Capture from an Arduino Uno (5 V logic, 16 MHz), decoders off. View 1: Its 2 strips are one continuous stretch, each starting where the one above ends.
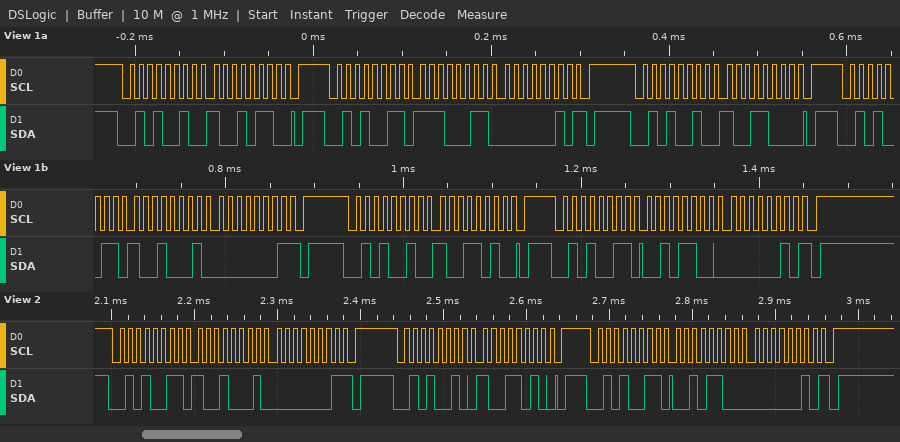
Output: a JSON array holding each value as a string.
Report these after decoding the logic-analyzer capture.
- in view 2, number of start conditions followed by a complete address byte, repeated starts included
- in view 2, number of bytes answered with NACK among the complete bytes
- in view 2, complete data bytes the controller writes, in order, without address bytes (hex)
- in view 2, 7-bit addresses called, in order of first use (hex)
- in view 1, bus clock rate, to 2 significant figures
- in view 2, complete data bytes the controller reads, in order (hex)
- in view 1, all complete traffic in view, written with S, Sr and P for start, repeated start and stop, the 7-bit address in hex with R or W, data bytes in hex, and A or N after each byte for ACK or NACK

["3", "2", "9A", "0x29", "100 kHz", "91 01 2C 02", "S 29W A 96 A P S 29R A E3 A 02 N P S 29W A 98 A P S 29R A 91 A 01 N P S 29W A 9A A P S 29R A 2C A 02 N P"]
